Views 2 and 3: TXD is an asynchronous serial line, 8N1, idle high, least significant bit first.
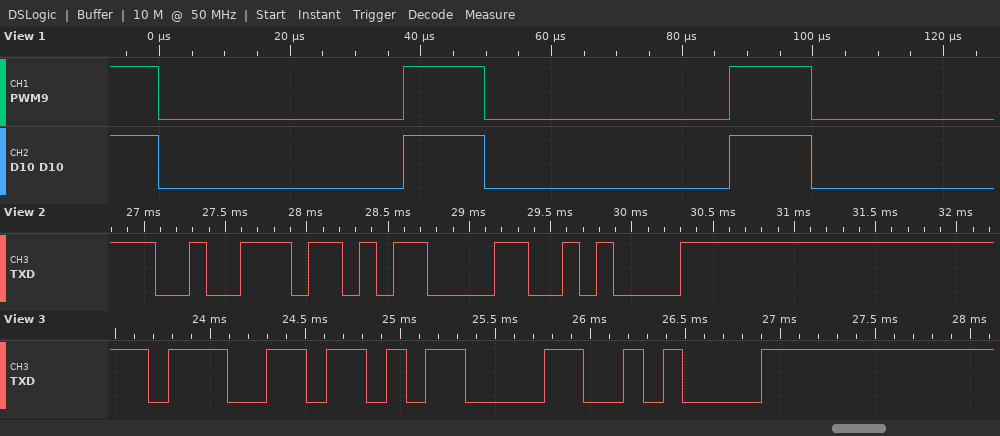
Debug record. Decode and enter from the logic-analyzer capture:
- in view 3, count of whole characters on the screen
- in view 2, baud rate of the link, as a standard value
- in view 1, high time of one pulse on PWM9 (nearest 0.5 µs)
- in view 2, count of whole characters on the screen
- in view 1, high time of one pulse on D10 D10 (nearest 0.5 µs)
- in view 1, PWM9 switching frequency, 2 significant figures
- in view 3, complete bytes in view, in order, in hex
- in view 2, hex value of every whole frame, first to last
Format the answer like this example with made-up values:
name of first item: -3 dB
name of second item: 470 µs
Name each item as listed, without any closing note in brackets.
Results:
in view 3, count of whole characters on the screen: 3
in view 2, baud rate of the link, as a standard value: 9600 baud
in view 1, high time of one pulse on PWM9: 12.5 µs
in view 2, count of whole characters on the screen: 3
in view 1, high time of one pulse on D10 D10: 12.5 µs
in view 1, PWM9 switching frequency, 2 significant figures: 20 kHz
in view 3, complete bytes in view, in order, in hex: 67 0D 0A
in view 2, hex value of every whole frame, first to last: 72 0D 0A
